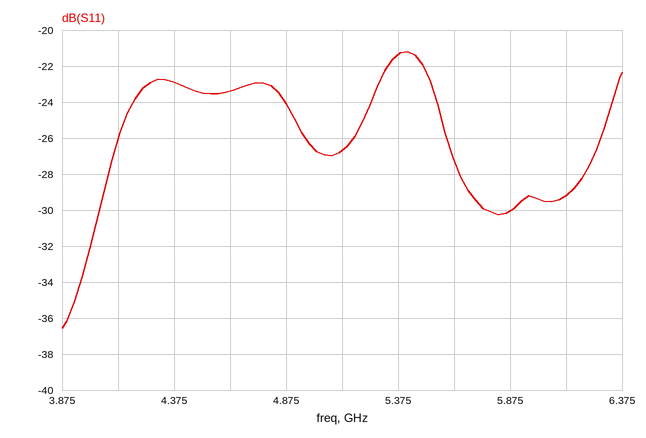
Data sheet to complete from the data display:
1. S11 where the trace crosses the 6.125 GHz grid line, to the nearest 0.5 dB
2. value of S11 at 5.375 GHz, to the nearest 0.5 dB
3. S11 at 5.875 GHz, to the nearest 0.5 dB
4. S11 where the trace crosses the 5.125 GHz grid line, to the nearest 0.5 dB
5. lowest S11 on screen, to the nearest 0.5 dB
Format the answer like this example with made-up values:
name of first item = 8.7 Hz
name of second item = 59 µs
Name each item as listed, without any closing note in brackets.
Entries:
S11 where the trace crosses the 6.125 GHz grid line, to the nearest 0.5 dB = -29.0 dB
value of S11 at 5.375 GHz, to the nearest 0.5 dB = -21.5 dB
S11 at 5.875 GHz, to the nearest 0.5 dB = -30.0 dB
S11 where the trace crosses the 5.125 GHz grid line, to the nearest 0.5 dB = -26.5 dB
lowest S11 on screen, to the nearest 0.5 dB = -36.5 dB
